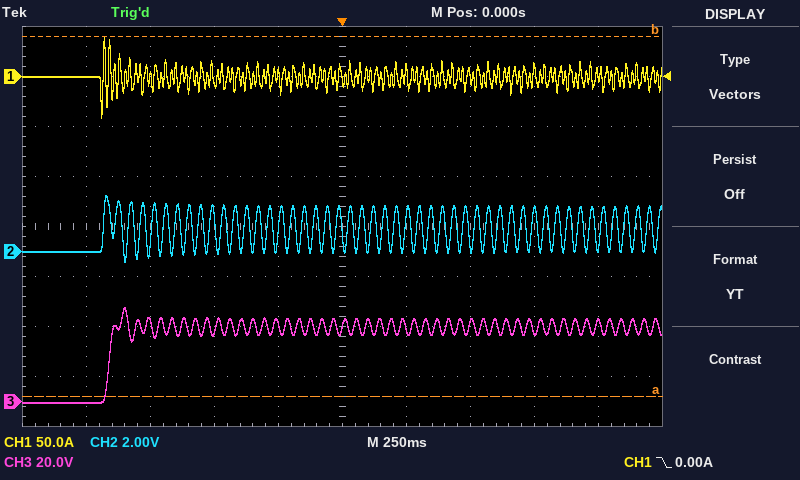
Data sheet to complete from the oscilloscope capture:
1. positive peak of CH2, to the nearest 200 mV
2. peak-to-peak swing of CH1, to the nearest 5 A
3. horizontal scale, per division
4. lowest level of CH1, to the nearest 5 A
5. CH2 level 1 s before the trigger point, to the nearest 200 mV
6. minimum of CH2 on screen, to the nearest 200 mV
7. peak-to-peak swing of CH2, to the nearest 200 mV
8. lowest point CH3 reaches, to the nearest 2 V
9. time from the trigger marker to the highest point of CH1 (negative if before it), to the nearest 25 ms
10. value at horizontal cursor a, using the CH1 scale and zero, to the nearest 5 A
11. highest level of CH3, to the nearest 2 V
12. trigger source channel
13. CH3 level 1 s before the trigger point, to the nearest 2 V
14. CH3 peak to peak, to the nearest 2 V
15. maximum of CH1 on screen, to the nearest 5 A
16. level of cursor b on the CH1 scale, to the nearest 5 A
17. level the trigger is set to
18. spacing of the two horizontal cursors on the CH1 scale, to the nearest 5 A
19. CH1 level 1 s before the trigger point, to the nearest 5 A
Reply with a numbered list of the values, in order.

1. 2.2 V
2. 80 A
3. 250 ms
4. -40 A
5. 0.0 V
6. -400 mV
7. 2.6 V
8. 0 V
9. -925 ms
10. -320 A
11. 38 V
12. CH1
13. 0 V
14. 38 V
15. 40 A
16. 40 A
17. 0.00 A
18. 360 A
19. 0 A
